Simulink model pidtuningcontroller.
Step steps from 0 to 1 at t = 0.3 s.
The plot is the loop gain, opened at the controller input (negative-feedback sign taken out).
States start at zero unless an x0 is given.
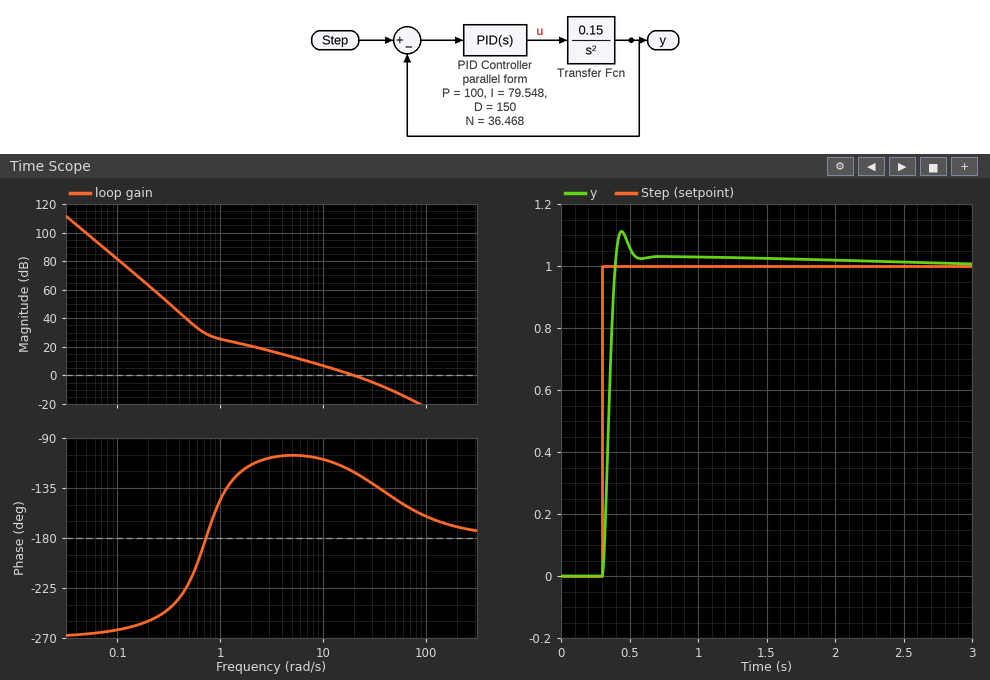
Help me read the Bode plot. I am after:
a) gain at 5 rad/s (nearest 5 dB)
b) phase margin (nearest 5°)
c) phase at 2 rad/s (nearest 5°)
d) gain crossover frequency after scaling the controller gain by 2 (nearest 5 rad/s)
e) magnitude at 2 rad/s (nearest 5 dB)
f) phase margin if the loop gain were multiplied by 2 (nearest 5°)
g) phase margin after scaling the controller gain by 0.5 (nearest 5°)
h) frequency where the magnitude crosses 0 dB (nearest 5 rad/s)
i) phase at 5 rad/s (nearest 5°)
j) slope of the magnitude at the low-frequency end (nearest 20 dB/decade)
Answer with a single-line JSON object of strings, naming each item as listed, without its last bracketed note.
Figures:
{"gain at 5 rad/s": "15 dB", "phase margin": "60°", "phase at 2 rad/s": "-115°", "gain crossover frequency after scaling the controller gain by 2": "35 rad/s", "magnitude at 2 rad/s": "20 dB", "phase margin if the loop gain were multiplied by 2": "45°", "phase margin after scaling the controller gain by 0.5": "70°", "frequency where the magnitude crosses 0 dB": "20 rad/s", "phase at 5 rad/s": "-105°", "slope of the magnitude at the low-frequency end": "-60 dB/decade"}
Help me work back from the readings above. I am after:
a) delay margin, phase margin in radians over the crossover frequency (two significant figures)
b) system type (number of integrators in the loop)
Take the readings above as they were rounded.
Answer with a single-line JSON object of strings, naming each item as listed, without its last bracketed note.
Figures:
{"delay margin, phase margin in radians over the crossover frequency": "0.052 s", "system type": "3"}
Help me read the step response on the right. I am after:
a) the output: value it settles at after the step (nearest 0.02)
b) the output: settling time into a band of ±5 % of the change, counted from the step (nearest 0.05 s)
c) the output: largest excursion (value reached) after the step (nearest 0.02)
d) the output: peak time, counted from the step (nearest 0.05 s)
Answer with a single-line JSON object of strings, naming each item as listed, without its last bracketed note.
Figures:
{"the output: value it settles at after the step": "1.00", "the output: settling time into a band of ±5 % of the change, counted from the step": "0.20 s", "the output: largest excursion (value reached) after the step": "1.12", "the output: peak time, counted from the step": "0.15 s"}
